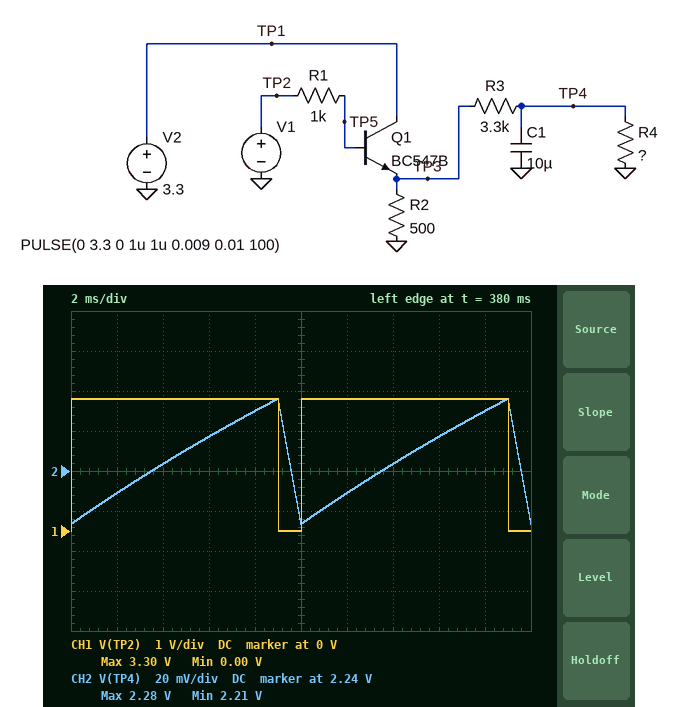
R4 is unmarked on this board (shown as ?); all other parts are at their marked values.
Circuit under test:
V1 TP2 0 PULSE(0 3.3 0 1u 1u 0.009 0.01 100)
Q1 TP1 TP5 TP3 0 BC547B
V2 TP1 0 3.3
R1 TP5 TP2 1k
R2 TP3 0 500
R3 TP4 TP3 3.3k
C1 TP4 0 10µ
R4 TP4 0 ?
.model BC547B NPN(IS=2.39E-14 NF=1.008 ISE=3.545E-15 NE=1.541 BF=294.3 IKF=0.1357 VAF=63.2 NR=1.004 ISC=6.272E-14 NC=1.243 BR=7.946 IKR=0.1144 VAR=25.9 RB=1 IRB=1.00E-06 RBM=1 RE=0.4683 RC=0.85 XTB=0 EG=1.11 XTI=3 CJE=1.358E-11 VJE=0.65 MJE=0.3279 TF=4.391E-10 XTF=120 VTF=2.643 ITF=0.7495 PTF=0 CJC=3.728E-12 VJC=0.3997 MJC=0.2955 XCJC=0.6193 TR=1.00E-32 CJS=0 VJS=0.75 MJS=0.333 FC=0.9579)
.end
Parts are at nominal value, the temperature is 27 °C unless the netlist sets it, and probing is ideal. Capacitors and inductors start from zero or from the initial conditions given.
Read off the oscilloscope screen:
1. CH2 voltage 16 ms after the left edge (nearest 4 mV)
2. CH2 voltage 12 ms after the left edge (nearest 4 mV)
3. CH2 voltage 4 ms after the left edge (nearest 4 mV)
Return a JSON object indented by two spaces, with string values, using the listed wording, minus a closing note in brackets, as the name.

{
  "CH2 voltage 16 ms after the left edge": "2.256 V",
  "CH2 voltage 12 ms after the left edge": "2.228 V",
  "CH2 voltage 4 ms after the left edge": "2.244 V"
}
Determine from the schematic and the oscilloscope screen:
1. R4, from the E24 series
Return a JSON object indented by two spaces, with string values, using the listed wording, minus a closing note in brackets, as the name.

{
  "R4, from the E24 series": "62 kΩ"
}
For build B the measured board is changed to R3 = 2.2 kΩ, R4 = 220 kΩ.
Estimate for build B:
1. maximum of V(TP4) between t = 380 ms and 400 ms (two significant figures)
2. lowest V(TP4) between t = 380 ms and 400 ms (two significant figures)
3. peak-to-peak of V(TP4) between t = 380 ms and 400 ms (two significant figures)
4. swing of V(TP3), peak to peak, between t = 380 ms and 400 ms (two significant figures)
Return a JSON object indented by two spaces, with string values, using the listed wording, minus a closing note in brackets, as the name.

{
  "maximum of V(TP4) between t = 380 ms and 400 ms": "2.4 V",
  "lowest V(TP4) between t = 380 ms and 400 ms": "2.3 V",
  "peak-to-peak of V(TP4) between t = 380 ms and 400 ms": "88 mV",
  "swing of V(TP3), peak to peak, between t = 380 ms and 400 ms": "2.2 V"
}
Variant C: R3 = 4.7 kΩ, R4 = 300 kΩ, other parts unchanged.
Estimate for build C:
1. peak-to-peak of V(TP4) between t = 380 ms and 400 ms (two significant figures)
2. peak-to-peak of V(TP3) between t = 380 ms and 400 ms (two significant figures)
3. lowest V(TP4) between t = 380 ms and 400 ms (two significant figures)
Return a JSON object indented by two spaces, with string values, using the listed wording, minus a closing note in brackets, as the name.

{
  "peak-to-peak of V(TP4) between t = 380 ms and 400 ms": "46 mV",
  "peak-to-peak of V(TP3) between t = 380 ms and 400 ms": "2.4 V",
  "lowest V(TP4) between t = 380 ms and 400 ms": "2.3 V"
}
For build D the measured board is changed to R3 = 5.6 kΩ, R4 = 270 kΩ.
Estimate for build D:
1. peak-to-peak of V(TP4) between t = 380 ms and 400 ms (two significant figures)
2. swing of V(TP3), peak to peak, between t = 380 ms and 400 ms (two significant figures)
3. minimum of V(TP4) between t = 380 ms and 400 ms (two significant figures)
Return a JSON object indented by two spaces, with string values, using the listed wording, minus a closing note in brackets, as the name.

{
  "peak-to-peak of V(TP4) between t = 380 ms and 400 ms": "39 mV",
  "swing of V(TP3), peak to peak, between t = 380 ms and 400 ms": "2.4 V",
  "minimum of V(TP4) between t = 380 ms and 400 ms": "2.3 V"
}
